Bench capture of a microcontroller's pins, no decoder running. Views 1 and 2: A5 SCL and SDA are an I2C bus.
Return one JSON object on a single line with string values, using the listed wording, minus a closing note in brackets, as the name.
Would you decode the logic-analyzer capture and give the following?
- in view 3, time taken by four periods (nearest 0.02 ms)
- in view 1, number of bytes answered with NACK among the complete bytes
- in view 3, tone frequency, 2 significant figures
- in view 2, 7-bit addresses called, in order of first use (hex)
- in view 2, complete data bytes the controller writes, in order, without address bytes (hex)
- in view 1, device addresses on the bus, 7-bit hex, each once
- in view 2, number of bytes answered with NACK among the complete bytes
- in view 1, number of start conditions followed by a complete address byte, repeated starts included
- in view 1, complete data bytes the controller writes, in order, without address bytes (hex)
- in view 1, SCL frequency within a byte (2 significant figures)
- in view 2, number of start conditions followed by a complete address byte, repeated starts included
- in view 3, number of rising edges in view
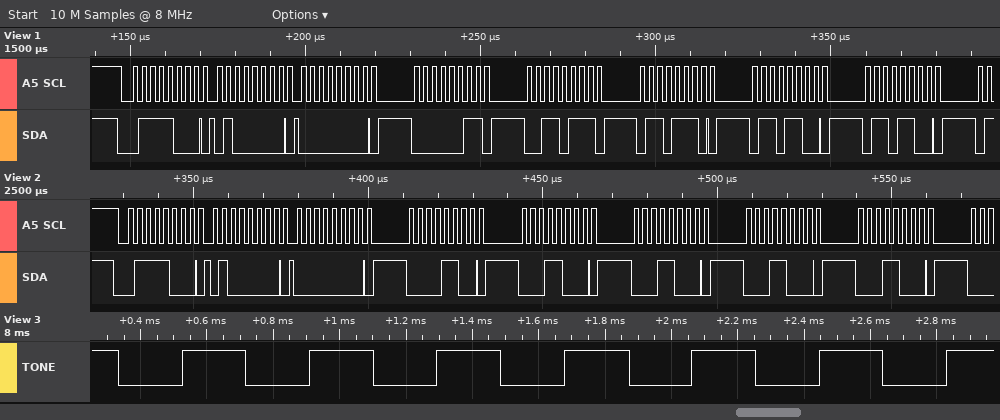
{"in view 3, time taken by four periods": "1.54 ms", "in view 1, number of bytes answered with NACK among the complete bytes": "0", "in view 3, tone frequency, 2 significant figures": "2.6 kHz", "in view 2, 7-bit addresses called, in order of first use": "0x3C", "in view 2, complete data bytes the controller writes, in order, without address bytes": "40 00 0C 18 18 18 18", "in view 1, device addresses on the bus, 7-bit hex, each once": "0x3C", "in view 2, number of bytes answered with NACK among the complete bytes": "0", "in view 1, number of start conditions followed by a complete address byte, repeated starts included": "1", "in view 1, complete data bytes the controller writes, in order, without address bytes": "40 00 03 37 6E 6C 6C", "in view 1, SCL frequency within a byte": "400 kHz", "in view 2, number of start conditions followed by a complete address byte, repeated starts included": "1", "in view 3, number of rising edges in view": "7"}
